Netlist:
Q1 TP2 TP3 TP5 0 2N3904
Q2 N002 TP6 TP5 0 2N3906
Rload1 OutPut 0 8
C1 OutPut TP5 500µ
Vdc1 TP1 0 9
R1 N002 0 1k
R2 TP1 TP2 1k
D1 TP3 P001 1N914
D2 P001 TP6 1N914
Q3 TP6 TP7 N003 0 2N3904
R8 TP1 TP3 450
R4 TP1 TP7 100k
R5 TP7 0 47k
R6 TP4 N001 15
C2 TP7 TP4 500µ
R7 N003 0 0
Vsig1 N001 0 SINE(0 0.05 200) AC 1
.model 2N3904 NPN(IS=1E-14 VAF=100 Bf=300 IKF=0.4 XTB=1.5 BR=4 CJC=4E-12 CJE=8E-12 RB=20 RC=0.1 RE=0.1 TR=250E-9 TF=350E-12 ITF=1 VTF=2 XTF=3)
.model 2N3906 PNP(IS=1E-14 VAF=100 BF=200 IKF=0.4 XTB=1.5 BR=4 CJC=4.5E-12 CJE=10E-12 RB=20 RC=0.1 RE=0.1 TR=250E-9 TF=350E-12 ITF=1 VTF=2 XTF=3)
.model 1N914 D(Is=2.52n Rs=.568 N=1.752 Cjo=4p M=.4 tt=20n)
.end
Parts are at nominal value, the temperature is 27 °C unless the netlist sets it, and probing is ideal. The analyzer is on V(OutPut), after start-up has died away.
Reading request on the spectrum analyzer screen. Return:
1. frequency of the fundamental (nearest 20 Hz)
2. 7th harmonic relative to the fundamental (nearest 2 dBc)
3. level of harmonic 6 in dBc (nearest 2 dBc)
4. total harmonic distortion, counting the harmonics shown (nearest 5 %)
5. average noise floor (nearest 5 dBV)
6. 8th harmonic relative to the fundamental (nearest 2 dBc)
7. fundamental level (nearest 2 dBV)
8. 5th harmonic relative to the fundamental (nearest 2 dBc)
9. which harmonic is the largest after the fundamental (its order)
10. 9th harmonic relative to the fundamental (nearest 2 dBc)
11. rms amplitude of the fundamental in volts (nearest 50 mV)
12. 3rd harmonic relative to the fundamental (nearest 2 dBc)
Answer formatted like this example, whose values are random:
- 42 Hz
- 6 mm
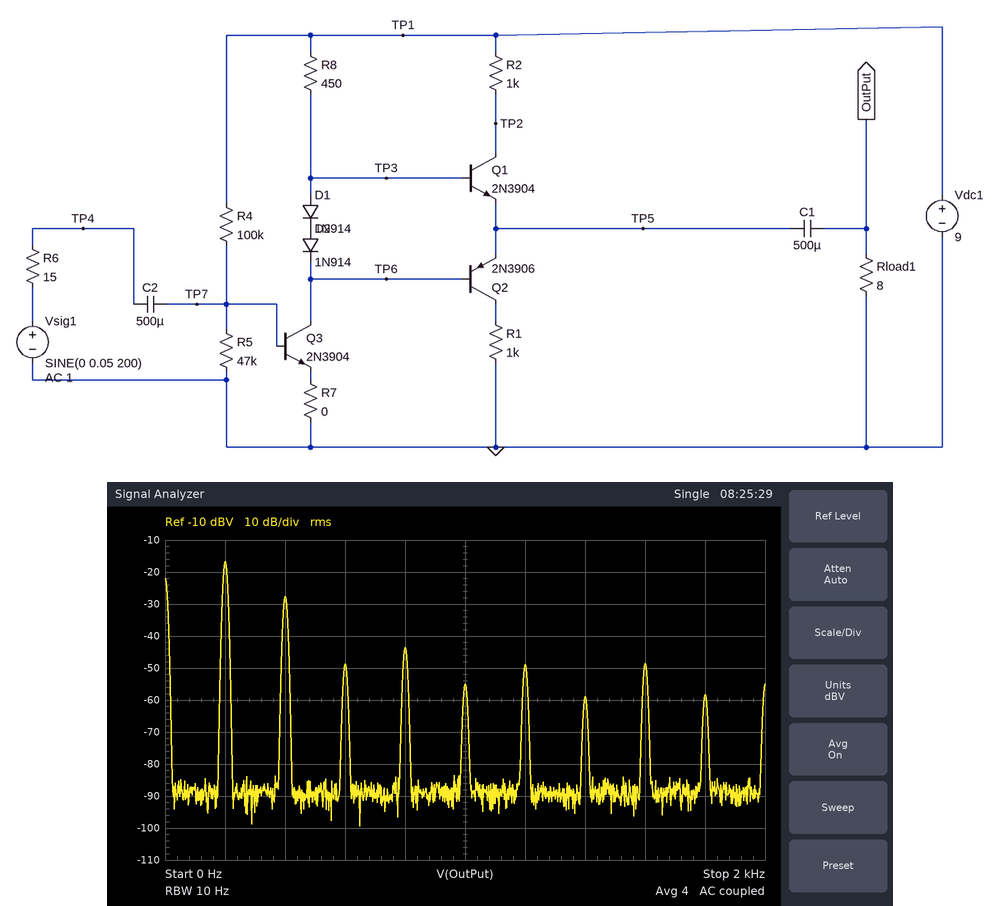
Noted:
- 200 Hz
- -42 dBc
- -32 dBc
- 30 %
- -90 dBV
- -32 dBc
- -16 dBV
- -38 dBc
- 2
- -42 dBc
- 150 mV
- -32 dBc
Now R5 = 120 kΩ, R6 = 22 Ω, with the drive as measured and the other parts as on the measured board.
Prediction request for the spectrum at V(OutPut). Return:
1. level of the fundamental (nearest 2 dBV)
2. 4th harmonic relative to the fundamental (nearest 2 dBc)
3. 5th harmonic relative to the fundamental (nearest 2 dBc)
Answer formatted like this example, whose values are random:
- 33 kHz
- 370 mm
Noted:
- -16 dBV
- -24 dBc
- -46 dBc
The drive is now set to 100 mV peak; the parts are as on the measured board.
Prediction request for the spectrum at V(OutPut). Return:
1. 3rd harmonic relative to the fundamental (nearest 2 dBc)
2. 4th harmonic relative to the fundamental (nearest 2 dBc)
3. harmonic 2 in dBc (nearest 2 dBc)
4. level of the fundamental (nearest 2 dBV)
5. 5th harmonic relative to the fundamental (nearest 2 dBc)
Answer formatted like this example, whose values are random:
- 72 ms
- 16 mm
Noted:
- -18 dBc
- -30 dBc
- -6 dBc
- -16 dBV
- -28 dBc
